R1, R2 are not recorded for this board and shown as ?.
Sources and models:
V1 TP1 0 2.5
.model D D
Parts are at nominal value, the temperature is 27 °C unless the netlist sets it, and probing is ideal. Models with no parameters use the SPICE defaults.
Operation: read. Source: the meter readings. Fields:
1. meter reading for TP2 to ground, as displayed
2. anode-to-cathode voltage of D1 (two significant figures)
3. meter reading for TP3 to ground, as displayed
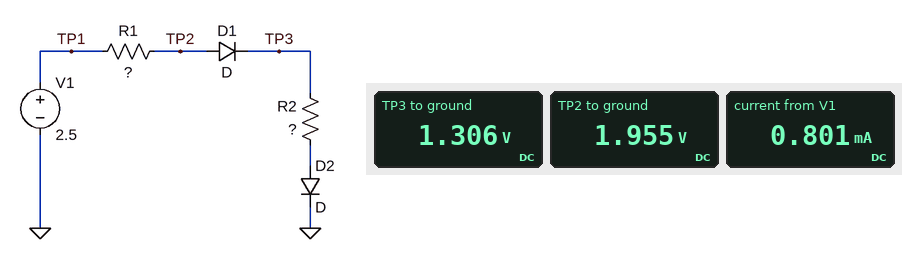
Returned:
1.955 V
650 mV
1.306 V
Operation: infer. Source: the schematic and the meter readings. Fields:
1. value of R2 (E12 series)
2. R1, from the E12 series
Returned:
820 Ω
680 Ω
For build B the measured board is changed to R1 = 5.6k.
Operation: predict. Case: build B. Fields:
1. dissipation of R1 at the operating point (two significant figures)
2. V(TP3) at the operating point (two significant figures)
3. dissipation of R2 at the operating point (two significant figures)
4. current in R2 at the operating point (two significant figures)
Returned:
220 µW
780 mV
32 µW
200 µA
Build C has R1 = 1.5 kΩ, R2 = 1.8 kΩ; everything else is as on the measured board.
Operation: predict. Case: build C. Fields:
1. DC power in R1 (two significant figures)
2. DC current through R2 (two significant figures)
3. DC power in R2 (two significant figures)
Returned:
210 µW
380 µA
250 µW
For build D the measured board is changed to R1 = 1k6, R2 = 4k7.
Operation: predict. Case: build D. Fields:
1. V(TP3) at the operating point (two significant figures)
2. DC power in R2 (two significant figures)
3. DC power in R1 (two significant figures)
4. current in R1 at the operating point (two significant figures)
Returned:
1.6 V
190 µW
65 µW
200 µA
